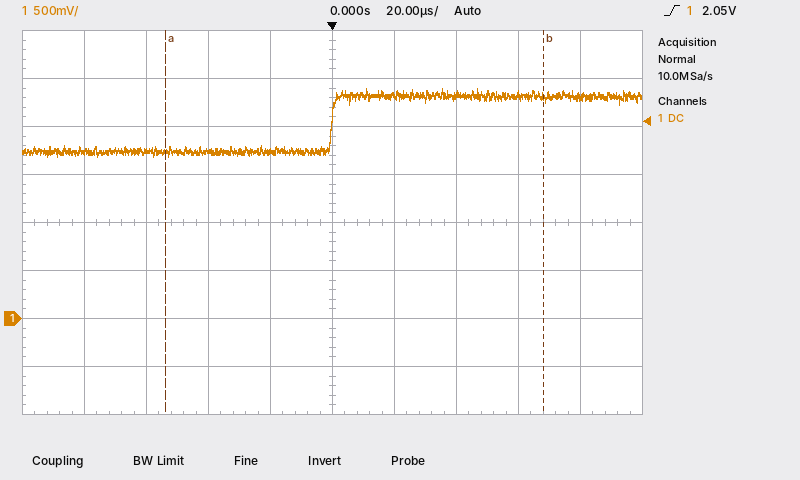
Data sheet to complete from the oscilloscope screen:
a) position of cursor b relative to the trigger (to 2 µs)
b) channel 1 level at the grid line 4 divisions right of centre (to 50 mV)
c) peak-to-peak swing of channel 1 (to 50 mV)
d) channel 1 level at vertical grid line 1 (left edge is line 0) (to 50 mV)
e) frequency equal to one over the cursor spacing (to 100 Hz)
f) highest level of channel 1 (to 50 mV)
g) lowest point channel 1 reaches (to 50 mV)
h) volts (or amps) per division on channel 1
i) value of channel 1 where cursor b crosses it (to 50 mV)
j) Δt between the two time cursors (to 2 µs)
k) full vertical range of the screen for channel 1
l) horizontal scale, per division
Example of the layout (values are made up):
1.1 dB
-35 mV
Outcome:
+68 µs
2.30 V
700 mV
1.75 V
8.2 kHz
2.40 V
1.70 V
500 mV
2.30 V
122 µs
4 V
20 µs
